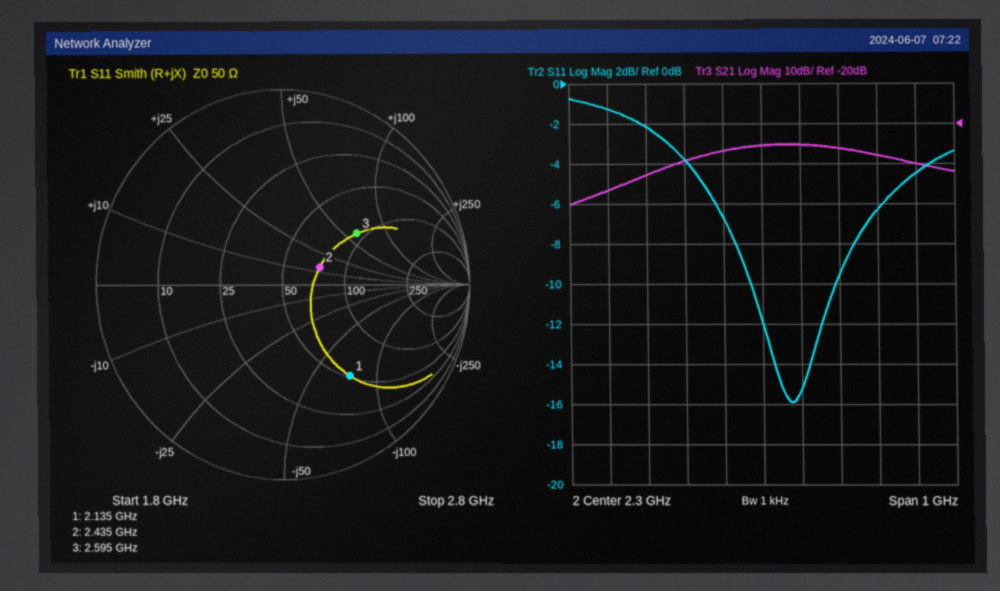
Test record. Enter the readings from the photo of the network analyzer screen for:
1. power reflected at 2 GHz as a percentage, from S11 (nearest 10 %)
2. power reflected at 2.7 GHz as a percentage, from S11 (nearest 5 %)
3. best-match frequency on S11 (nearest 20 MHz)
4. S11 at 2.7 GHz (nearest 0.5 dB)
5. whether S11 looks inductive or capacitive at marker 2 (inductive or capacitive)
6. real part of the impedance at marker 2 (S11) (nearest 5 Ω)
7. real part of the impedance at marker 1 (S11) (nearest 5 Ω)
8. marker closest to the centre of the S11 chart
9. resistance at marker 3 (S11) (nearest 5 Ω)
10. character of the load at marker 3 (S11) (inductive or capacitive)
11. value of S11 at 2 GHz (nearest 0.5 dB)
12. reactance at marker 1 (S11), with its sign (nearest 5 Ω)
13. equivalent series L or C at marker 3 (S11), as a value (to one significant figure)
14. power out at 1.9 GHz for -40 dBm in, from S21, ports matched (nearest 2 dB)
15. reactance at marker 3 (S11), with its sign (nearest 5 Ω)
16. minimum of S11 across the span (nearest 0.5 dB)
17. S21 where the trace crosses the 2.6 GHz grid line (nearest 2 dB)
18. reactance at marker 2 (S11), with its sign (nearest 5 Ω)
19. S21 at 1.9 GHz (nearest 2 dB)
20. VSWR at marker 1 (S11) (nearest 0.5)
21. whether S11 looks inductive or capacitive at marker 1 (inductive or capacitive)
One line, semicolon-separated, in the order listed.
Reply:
60 %; 35 %; 2.38 GHz; -4.5 dB; inductive; 75 Ω; 50 Ω; marker 2; 90 Ω; inductive; -2.0 dB; -75 Ω; 4 nH; -76 dBm; +60 Ω; -16.0 dB; -28 dB; +15 Ω; -36 dB; 4.0; capacitive
